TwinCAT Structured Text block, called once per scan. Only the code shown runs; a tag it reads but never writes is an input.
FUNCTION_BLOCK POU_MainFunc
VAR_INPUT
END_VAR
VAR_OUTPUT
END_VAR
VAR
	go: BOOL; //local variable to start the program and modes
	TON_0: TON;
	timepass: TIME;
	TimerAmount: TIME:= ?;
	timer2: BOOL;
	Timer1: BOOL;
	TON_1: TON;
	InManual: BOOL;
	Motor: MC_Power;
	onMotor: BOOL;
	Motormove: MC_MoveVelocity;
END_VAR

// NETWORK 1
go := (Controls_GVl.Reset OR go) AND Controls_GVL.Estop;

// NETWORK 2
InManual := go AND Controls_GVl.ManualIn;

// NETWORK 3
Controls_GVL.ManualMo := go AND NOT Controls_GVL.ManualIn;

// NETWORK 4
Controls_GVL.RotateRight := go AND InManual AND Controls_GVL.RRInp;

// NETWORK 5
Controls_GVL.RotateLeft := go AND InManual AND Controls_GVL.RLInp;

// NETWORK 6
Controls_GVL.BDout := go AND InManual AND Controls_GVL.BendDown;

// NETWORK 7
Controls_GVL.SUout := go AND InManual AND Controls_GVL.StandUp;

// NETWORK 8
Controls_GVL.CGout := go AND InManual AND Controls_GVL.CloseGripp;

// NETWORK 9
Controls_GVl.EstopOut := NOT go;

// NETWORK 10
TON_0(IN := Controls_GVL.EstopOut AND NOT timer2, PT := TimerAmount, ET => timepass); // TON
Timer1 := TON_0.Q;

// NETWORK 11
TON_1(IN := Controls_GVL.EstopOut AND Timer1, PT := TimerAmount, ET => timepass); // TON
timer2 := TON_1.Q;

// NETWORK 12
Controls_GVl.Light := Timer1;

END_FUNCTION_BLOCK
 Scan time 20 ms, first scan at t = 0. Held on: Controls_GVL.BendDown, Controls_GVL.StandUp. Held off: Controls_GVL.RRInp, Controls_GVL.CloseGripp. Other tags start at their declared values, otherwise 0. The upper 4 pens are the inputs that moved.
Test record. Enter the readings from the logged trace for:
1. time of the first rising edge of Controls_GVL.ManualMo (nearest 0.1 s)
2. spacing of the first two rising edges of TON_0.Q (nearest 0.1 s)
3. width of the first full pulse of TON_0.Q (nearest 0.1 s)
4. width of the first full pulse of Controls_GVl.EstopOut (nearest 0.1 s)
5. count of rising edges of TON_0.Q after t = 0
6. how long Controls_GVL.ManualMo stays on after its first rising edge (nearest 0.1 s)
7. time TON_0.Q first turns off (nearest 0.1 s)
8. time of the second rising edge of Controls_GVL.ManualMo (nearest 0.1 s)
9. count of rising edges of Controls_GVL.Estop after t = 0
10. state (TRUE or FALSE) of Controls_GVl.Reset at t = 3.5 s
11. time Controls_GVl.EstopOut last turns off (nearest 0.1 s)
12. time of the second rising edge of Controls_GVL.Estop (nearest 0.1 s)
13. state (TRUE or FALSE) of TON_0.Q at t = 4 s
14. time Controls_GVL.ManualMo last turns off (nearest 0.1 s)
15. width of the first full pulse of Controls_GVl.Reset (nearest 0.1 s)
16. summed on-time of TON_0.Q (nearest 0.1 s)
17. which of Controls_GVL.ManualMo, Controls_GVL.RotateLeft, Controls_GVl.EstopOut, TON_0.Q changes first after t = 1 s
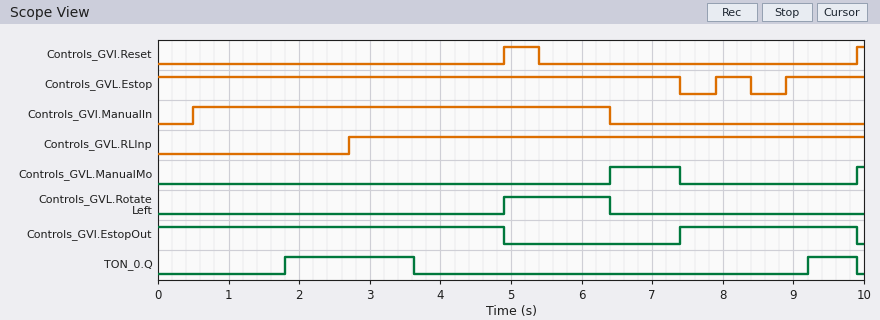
6.4 s
7.4 s
1.8 s
2.5 s
2
1.0 s
3.6 s
9.9 s
2
FALSE
9.9 s
8.9 s
FALSE
7.4 s
0.5 s
2.5 s
TON_0.Q
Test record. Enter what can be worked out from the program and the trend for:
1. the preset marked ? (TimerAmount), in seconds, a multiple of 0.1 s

1.8 s
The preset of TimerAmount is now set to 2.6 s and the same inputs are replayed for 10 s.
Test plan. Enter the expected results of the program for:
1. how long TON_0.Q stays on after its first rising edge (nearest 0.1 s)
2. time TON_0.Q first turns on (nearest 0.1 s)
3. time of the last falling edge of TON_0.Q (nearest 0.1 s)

2.3 s
2.6 s
4.9 s
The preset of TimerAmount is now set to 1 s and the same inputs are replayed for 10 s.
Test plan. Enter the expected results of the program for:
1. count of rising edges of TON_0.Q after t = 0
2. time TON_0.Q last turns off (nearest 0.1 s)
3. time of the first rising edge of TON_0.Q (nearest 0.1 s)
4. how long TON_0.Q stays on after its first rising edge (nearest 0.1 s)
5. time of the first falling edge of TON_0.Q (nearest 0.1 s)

3
9.4 s
1.0 s
1.0 s
2.0 s
